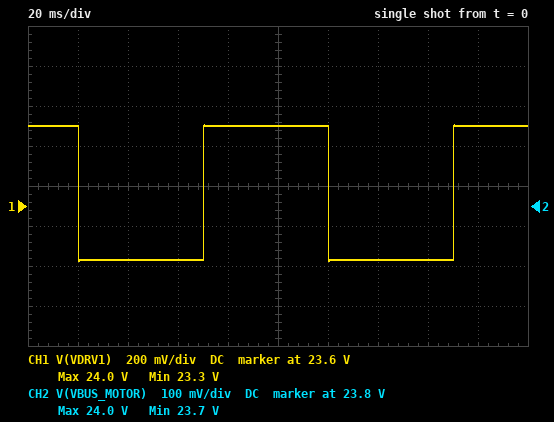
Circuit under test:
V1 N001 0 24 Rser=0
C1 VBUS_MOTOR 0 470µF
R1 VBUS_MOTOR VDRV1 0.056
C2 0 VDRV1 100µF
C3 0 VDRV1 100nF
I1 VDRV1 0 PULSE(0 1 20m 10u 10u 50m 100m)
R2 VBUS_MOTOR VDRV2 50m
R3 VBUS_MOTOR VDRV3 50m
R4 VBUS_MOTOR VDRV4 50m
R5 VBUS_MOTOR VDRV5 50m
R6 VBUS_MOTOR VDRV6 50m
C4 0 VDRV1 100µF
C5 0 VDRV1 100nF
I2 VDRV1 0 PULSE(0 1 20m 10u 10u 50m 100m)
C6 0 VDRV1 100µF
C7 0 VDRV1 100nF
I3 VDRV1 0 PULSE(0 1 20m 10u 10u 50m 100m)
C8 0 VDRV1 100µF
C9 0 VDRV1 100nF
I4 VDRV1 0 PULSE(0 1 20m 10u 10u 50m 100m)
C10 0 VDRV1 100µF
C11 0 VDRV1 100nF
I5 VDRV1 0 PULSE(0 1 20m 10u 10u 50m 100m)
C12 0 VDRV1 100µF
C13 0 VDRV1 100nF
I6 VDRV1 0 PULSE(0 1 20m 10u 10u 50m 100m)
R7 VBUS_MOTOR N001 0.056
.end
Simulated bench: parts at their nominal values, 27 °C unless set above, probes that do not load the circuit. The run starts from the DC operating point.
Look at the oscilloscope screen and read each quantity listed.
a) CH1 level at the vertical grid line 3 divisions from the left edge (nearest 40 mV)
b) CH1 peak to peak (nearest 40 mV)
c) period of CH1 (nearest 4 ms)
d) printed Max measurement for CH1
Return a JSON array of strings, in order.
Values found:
["23.32 V", "680 mV", "100 ms", "24.0 V"]
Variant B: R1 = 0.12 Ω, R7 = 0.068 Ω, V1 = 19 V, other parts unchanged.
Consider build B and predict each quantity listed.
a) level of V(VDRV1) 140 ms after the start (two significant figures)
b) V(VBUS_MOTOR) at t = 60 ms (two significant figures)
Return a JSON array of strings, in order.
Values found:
["18 V", "19 V"]
